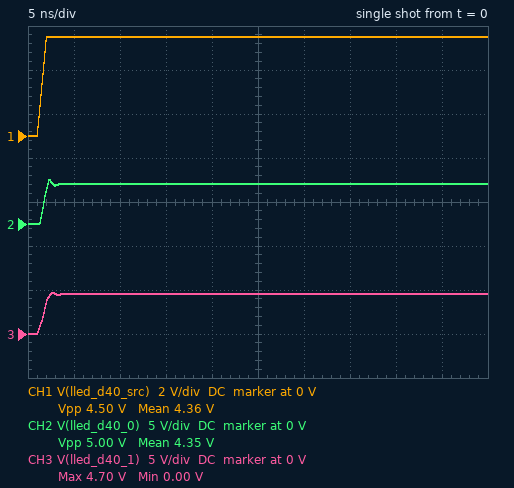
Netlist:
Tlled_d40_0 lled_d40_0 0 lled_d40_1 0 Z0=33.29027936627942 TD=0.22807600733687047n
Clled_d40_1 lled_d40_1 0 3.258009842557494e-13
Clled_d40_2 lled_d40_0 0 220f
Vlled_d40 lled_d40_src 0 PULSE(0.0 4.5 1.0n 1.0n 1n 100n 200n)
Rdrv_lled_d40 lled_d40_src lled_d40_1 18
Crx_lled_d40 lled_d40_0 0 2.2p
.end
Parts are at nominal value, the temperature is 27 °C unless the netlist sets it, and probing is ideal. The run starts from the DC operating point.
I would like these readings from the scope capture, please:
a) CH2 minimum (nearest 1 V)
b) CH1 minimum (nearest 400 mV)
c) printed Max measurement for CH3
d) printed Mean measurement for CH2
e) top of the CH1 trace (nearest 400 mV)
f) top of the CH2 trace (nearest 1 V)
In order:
0 V
0 V
4.70 V
4.35 V
4.4 V
5 V
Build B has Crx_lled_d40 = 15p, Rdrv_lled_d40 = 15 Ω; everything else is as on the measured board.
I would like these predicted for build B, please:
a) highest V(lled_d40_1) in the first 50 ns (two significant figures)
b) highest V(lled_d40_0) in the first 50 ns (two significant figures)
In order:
4.9 V
5.3 V
